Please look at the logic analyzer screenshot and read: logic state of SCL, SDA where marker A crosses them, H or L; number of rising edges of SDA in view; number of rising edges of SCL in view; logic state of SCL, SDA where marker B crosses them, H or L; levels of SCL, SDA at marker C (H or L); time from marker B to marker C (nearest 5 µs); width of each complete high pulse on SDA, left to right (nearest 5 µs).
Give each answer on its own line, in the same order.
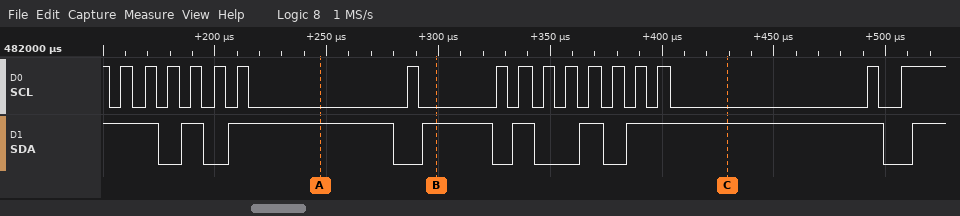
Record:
SCL=L, SDA=H
7
17
SCL=L, SDA=H
SCL=L, SDA=H
130 µs
10 µs, 75 µs, 30 µs, 10 µs, 10 µs, 115 µs
